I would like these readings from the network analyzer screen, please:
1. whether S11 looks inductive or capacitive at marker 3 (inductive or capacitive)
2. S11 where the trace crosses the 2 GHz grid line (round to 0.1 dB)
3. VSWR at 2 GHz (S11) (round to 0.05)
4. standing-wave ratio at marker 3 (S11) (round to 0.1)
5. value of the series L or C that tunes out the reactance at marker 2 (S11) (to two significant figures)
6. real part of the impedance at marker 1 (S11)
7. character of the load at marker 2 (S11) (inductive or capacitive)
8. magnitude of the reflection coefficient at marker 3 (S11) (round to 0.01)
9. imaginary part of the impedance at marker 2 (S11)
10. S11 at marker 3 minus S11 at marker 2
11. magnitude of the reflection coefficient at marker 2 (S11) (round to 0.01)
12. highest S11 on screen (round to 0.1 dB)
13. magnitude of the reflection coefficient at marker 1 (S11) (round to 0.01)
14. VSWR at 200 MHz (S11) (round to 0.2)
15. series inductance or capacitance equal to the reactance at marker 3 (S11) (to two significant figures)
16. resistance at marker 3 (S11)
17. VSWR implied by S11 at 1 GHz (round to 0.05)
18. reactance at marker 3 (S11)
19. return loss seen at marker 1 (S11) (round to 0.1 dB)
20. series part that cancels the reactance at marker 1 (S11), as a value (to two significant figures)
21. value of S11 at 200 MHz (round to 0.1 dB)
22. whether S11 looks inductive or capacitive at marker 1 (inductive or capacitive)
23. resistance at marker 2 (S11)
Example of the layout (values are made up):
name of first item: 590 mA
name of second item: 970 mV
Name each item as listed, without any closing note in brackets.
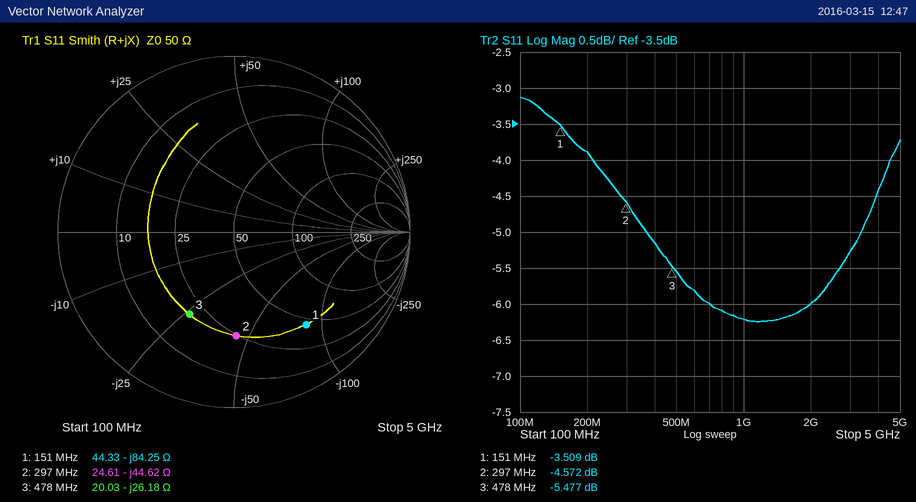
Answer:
whether S11 looks inductive or capacitive at marker 3: capacitive
S11 where the trace crosses the 2 GHz grid line: -6.0 dB
VSWR at 2 GHz (S11): 3.00
standing-wave ratio at marker 3 (S11): 3.3
value of the series L or C that tunes out the reactance at marker 2 (S11): 24 nH
real part of the impedance at marker 1: 44.33 Ω
character of the load at marker 2 (S11): capacitive
magnitude of the reflection coefficient at marker 3 (S11): 0.53
imaginary part of the impedance at marker 2: -44.62 Ω
S11 at marker 3 minus S11 at marker 2: -0.905 dB
magnitude of the reflection coefficient at marker 2 (S11): 0.59
highest S11 on screen: -3.1 dB
magnitude of the reflection coefficient at marker 1 (S11): 0.67
VSWR at 200 MHz (S11): 4.6
series inductance or capacitance equal to the reactance at marker 3 (S11): 13 pF
resistance at marker 3: 20.03 Ω
VSWR implied by S11 at 1 GHz: 2.90
reactance at marker 3: -26.18 Ω
return loss seen at marker 1 (S11): 3.5 dB
series part that cancels the reactance at marker 1 (S11), as a value: 89 nH
value of S11 at 200 MHz: -3.9 dB
whether S11 looks inductive or capacitive at marker 1: capacitive
resistance at marker 2: 24.61 Ω
